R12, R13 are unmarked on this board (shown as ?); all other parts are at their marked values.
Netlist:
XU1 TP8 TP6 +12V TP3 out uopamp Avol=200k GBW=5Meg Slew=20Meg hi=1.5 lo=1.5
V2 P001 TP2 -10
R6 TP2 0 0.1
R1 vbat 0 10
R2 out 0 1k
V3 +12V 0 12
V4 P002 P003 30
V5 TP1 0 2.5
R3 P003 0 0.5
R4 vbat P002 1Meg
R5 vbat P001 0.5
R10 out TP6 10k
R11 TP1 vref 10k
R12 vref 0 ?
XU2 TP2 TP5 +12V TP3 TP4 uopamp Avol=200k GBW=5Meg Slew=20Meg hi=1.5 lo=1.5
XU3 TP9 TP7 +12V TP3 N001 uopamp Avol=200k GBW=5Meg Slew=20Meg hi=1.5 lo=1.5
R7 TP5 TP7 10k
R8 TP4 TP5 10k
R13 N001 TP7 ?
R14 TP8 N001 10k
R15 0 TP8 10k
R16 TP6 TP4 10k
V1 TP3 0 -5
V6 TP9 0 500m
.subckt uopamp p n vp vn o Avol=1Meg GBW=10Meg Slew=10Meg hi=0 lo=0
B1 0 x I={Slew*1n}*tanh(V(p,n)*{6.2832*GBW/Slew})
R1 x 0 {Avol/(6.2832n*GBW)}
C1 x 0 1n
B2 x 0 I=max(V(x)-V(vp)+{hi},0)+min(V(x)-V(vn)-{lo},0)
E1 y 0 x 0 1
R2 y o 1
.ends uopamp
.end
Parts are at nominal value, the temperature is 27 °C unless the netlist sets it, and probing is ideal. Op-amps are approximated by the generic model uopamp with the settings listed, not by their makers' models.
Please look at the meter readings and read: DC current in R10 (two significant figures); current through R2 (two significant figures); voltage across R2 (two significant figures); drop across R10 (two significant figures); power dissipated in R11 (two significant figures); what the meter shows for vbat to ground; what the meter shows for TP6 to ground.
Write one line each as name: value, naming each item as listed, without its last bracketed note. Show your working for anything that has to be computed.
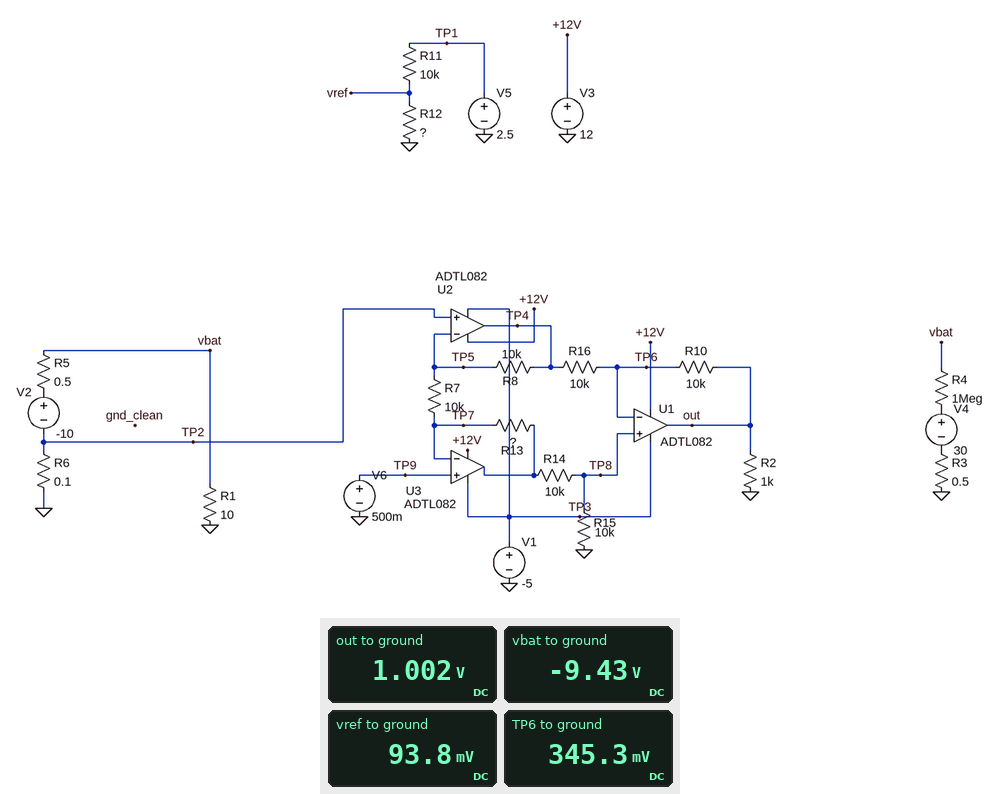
DC current in R10: (1.002 V - 345.3 mV) / 10 kΩ = 66 µA
current through R2: (1.002 V) / 1 kΩ = 1.0 mA
voltage across R2: 1.002 V = 1.0 V
drop across R10: 1.002 V - 345.3 mV = 660 mV
power dissipated in R11: (2.5 V - 93.8 mV)^2 / 10 kΩ = 580 µW
what the meter shows for vbat to ground: -9.43 V
what the meter shows for TP6 to ground: 345.3 mV
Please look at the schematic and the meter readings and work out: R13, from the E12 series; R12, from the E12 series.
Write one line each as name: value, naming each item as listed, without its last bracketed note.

R13, from the E12 series: 4.7 kΩ
R12, from the E12 series: 390 Ω
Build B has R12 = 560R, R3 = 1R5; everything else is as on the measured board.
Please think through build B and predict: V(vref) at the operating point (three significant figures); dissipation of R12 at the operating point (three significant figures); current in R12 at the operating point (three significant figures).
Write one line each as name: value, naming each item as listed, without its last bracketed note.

V(vref) at the operating point: 133 mV
dissipation of R12 at the operating point: 31.4 µW
current in R12 at the operating point: 237 µA
